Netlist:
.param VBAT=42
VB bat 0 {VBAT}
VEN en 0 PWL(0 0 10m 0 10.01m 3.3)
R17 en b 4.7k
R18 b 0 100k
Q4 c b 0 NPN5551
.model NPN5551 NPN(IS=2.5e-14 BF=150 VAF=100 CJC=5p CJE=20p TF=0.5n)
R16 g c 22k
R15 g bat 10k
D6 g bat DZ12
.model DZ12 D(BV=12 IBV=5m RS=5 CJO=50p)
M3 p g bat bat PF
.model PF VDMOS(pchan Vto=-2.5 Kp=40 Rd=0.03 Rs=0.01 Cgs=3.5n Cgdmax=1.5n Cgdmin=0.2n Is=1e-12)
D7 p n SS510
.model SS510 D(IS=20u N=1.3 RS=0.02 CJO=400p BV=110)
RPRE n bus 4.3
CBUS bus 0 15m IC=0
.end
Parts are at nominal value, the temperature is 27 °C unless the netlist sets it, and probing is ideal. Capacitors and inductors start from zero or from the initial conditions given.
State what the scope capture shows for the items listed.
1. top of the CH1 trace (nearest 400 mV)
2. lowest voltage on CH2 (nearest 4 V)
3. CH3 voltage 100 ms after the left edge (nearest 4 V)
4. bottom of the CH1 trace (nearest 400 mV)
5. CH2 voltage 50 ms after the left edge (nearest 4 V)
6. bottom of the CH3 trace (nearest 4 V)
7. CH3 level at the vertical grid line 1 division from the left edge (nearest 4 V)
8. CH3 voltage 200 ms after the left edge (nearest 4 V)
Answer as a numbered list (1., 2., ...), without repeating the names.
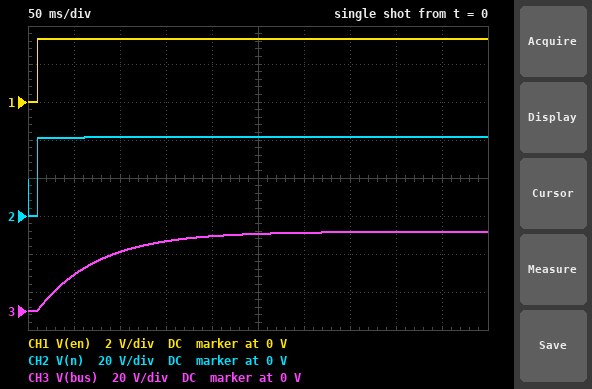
1. 3.2 V
2. 0 V
3. 32 V
4. 0 V
5. 40 V
6. 0 V
7. 20 V
8. 40 V
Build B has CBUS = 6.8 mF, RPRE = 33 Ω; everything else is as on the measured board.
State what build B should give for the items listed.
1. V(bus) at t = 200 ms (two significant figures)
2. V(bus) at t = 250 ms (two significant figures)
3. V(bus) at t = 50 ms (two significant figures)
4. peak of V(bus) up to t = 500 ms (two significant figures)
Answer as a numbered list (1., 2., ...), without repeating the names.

1. 24 V
2. 27 V
3. 6.8 V
4. 37 V
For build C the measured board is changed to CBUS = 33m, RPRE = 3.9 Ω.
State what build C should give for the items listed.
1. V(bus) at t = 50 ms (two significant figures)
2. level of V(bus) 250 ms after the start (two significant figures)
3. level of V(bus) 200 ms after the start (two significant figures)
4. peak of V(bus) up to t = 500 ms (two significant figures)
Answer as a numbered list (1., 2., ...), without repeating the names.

1. 11 V
2. 35 V
3. 32 V
4. 41 V
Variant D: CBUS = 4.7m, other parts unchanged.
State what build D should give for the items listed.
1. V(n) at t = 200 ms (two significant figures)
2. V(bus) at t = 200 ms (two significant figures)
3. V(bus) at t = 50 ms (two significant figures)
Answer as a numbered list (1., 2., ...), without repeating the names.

1. 42 V
2. 42 V
3. 36 V
